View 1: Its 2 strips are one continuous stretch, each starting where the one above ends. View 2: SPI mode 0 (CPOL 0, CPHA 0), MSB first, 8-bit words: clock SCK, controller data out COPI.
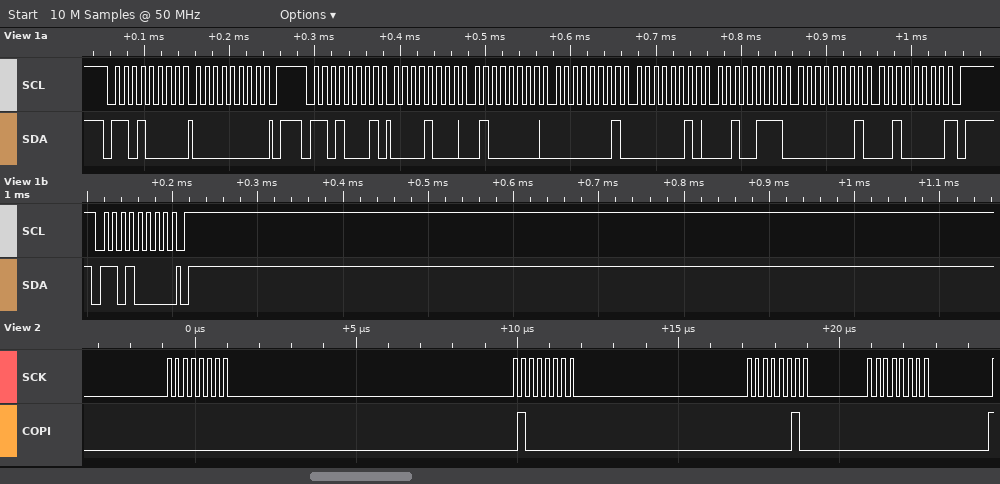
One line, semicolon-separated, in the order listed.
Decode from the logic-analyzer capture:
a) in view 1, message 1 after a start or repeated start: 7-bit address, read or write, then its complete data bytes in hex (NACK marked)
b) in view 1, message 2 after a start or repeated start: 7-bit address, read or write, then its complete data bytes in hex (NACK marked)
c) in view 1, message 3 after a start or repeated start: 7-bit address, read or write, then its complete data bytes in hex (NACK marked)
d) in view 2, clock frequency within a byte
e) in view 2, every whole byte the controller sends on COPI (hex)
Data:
0x68 write: 00; 0x68 read: 08 40 01 02 27 01 20 NACK; 0x68 write; 4 MHz; 00 40 02 00
